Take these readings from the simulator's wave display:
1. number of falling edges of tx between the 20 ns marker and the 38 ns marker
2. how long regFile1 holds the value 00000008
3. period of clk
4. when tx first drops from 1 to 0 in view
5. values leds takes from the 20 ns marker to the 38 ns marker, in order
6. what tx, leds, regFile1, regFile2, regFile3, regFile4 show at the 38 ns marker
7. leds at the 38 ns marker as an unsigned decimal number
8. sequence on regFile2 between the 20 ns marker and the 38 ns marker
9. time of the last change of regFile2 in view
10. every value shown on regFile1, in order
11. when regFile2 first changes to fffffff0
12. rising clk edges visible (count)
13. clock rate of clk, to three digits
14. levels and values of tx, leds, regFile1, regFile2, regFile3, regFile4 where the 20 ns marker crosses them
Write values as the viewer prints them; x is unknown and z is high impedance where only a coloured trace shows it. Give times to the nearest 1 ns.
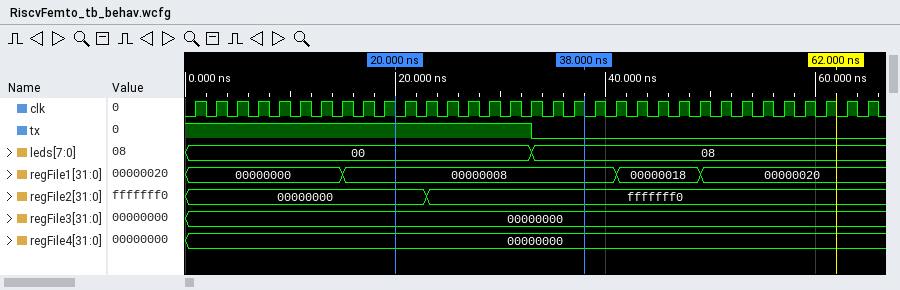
1
26 ns
2 ns
33 ns
00, 08
tx=0, leds=08, regFile1=00000008, regFile2=fffffff0, regFile3=00000000, regFile4=00000000
8
00000000, fffffff0
23 ns
00000000, 00000008, 00000018, 00000020
23 ns
33
500 MHz
tx=1, leds=00, regFile1=00000008, regFile2=00000000, regFile3=00000000, regFile4=00000000
